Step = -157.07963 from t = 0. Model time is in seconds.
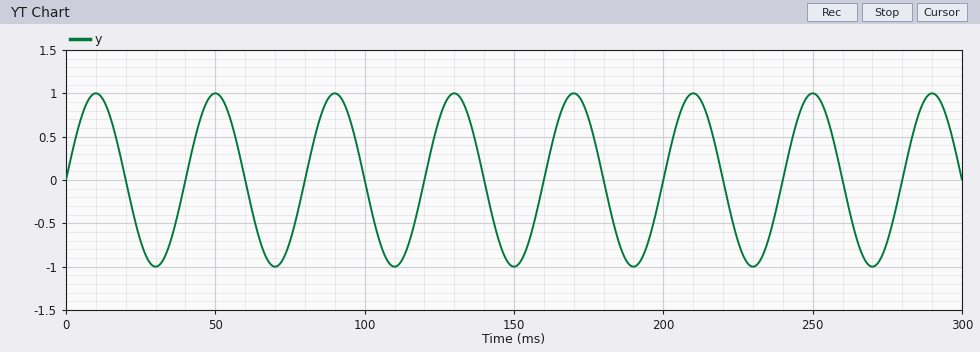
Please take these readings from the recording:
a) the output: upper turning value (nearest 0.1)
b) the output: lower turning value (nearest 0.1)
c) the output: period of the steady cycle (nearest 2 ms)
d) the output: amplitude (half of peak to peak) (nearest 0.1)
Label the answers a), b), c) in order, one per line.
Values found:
a) 1.0
b) -1.0
c) 40 ms
d) 1.0
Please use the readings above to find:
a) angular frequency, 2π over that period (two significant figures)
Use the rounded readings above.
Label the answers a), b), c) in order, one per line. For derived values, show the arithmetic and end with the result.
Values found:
a) 2π / 40 = 0.16 rad/ms
